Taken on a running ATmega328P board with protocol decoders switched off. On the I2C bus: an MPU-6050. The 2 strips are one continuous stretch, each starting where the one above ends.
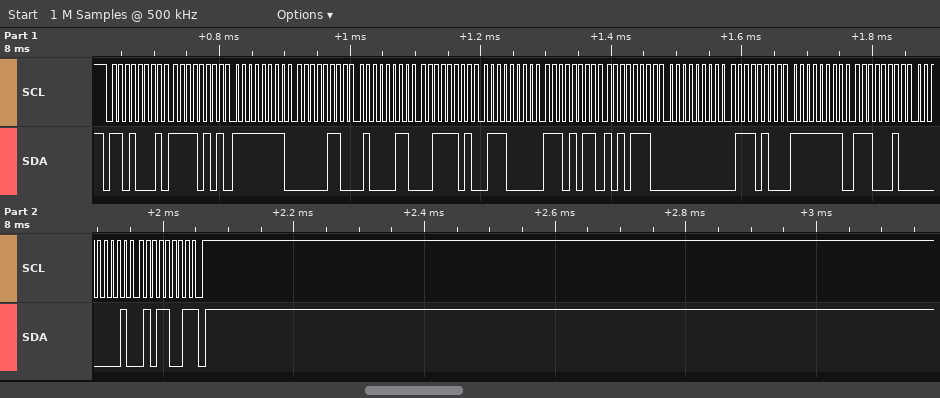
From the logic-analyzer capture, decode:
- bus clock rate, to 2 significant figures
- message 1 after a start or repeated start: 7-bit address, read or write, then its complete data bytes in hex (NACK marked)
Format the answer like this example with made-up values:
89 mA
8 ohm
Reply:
100 kHz
0x68 read: F5 FF 06 43 3D 70 EB AE 00 74 FF E2 01 59 NACK
